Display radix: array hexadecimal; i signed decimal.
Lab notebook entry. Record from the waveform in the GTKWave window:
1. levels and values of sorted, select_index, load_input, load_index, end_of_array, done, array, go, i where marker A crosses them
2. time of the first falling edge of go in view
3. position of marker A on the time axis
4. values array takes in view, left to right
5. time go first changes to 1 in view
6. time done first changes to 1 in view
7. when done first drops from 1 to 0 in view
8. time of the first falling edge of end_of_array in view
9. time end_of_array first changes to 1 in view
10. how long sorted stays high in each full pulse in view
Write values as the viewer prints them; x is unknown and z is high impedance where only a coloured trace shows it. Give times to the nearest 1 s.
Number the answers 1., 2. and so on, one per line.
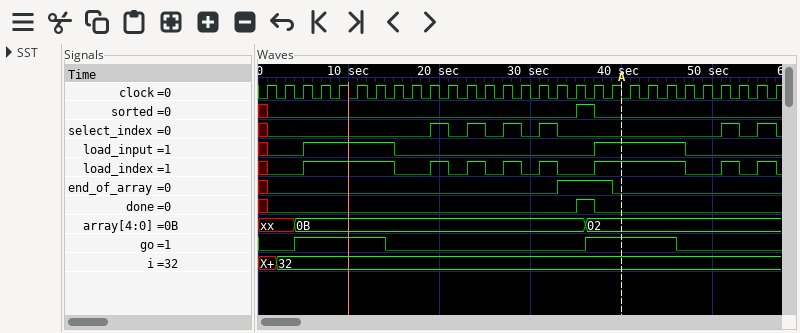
1. sorted=0, select_index=0, load_input=1, load_index=1, end_of_array=0, done=0, array=02, go=1, i=32
2. 14 s
3. 40 s
4. xx, 0B, 02
5. 4 s
6. 35 s
7. 37 s
8. 39 s
9. 33 s
10. 2 s
